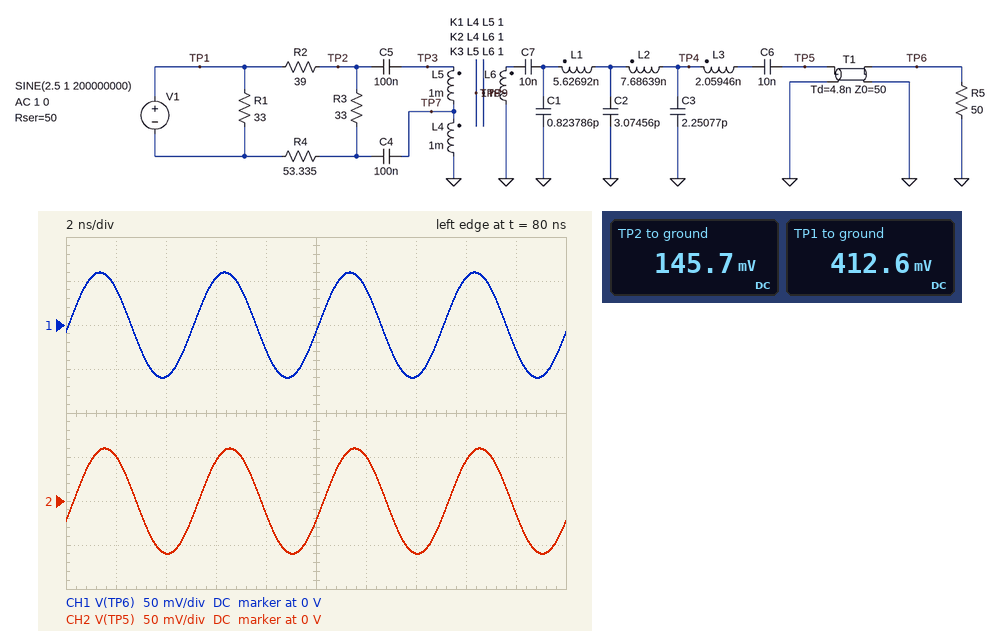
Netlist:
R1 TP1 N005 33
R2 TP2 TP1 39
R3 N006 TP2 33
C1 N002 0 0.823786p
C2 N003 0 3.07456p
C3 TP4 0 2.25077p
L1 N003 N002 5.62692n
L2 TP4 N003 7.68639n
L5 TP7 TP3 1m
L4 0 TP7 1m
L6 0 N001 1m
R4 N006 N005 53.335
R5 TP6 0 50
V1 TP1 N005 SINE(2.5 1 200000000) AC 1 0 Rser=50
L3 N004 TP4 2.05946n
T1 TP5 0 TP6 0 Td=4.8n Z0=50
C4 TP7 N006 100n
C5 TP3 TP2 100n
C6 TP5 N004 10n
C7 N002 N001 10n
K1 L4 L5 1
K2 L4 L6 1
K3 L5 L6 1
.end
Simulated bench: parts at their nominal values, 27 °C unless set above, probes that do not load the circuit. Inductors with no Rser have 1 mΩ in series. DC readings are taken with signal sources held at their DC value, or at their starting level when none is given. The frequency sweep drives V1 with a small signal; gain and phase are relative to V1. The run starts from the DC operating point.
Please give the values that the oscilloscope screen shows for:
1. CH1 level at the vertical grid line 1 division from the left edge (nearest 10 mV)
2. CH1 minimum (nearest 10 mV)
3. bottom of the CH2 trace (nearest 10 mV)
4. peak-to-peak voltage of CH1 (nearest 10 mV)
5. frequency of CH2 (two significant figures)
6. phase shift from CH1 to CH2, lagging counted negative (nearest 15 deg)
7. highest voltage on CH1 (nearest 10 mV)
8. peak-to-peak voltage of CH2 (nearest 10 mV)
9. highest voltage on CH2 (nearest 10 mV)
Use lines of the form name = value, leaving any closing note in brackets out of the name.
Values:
CH1 level at the vertical grid line 1 division from the left edge = 40 mV
CH1 minimum = -60 mV
bottom of the CH2 trace = -60 mV
peak-to-peak voltage of CH1 = 120 mV
frequency of CH2 = 200 MHz
phase shift from CH1 to CH2, lagging counted negative = -15 deg
highest voltage on CH1 = 60 mV
peak-to-peak voltage of CH2 = 120 mV
highest voltage on CH2 = 60 mV
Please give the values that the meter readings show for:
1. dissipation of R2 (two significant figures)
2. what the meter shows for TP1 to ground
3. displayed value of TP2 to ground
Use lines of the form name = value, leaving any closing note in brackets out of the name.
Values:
dissipation of R2 = 1.8 mW
what the meter shows for TP1 to ground = 412.6 mV
displayed value of TP2 to ground = 145.7 mV
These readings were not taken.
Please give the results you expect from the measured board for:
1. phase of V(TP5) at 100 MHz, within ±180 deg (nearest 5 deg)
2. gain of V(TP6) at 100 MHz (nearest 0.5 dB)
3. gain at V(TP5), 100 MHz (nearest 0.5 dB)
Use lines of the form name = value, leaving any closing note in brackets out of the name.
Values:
phase of V(TP5) at 100 MHz, within ±180 deg = -10 deg
gain of V(TP6) at 100 MHz = -24.5 dB
gain at V(TP5), 100 MHz = -24.5 dB
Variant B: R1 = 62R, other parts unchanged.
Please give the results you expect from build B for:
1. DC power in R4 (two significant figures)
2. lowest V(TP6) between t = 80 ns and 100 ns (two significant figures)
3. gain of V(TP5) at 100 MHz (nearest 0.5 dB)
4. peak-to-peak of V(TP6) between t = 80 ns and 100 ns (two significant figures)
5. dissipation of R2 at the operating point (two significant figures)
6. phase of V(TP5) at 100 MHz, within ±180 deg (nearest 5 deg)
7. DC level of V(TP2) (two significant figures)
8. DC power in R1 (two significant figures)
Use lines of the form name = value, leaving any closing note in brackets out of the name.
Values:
DC power in R4 = 4.4 mW
lowest V(TP6) between t = 80 ns and 100 ns = -79 mV
gain of V(TP5) at 100 MHz = -22.0 dB
peak-to-peak of V(TP6) between t = 80 ns and 100 ns = 160 mV
dissipation of R2 at the operating point = 3.2 mW
phase of V(TP5) at 100 MHz, within ±180 deg = -10 deg
DC level of V(TP2) = 190 mV
DC power in R1 = 21 mW
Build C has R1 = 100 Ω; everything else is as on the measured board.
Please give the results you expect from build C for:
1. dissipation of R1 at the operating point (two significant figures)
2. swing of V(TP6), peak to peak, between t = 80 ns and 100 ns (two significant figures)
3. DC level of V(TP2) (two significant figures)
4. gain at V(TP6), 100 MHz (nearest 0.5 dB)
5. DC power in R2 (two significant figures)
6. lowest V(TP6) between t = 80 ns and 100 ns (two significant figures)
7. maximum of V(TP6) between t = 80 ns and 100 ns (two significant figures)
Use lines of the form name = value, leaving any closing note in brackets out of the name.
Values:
dissipation of R1 at the operating point = 17 mW
swing of V(TP6), peak to peak, between t = 80 ns and 100 ns = 180 mV
DC level of V(TP2) = 220 mV
gain at V(TP6), 100 MHz = -21.0 dB
DC power in R2 = 4.3 mW
lowest V(TP6) between t = 80 ns and 100 ns = -91 mV
maximum of V(TP6) between t = 80 ns and 100 ns = 91 mV
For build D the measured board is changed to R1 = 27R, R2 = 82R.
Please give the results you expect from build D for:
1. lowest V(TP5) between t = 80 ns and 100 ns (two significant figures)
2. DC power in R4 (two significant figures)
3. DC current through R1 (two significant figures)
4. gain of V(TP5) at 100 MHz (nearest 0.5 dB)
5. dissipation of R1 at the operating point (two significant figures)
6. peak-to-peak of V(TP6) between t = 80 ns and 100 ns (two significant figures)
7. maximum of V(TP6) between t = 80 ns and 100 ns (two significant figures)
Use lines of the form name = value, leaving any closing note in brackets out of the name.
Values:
lowest V(TP5) between t = 80 ns and 100 ns = -40 mV
DC power in R4 = 1.2 mW
DC current through R1 = 29 mA
gain of V(TP5) at 100 MHz = -28.0 dB
dissipation of R1 at the operating point = 23 mW
peak-to-peak of V(TP6) between t = 80 ns and 100 ns = 81 mV
maximum of V(TP6) between t = 80 ns and 100 ns = 40 mV
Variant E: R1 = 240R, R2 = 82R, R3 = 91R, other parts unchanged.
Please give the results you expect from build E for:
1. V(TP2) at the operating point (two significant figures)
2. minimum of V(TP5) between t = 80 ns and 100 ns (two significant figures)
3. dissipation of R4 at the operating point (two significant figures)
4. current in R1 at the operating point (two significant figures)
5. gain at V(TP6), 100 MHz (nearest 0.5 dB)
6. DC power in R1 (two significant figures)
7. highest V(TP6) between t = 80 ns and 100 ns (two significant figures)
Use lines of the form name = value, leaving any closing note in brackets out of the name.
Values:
V(TP2) at the operating point = 300 mV
minimum of V(TP5) between t = 80 ns and 100 ns = -130 mV
dissipation of R4 at the operating point = 3.2 mW
current in R1 at the operating point = 7.3 mA
gain at V(TP6), 100 MHz = -18.0 dB
DC power in R1 = 13 mW
highest V(TP6) between t = 80 ns and 100 ns = 130 mV
